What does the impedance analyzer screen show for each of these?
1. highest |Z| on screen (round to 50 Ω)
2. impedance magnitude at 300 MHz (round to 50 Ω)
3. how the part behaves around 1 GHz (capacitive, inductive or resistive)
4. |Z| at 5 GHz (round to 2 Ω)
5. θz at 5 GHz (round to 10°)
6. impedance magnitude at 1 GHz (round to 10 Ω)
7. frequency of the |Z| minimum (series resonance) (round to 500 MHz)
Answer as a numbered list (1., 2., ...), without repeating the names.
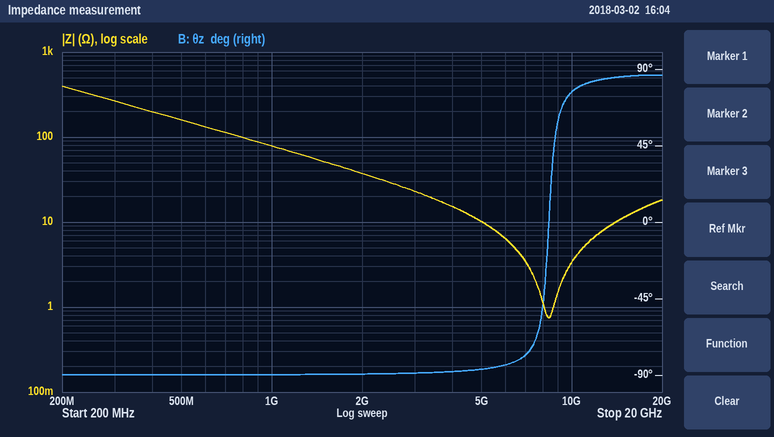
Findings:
1. 400 Ω
2. 250 Ω
3. capacitive
4. 10 Ω
5. -90°
6. 80 Ω
7. 8.5 GHz
